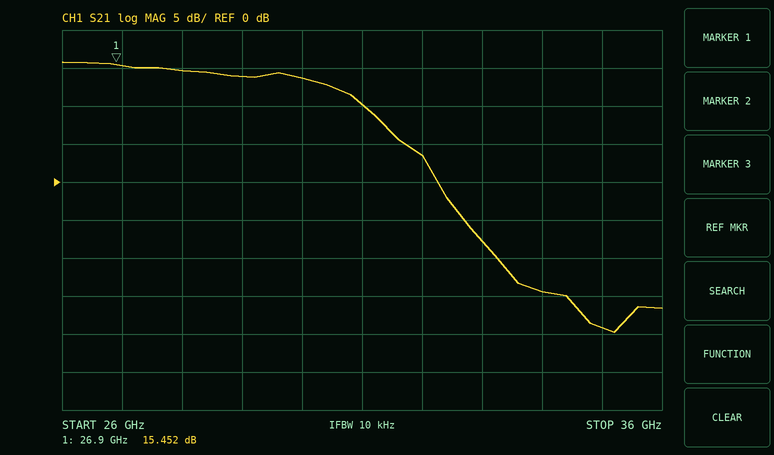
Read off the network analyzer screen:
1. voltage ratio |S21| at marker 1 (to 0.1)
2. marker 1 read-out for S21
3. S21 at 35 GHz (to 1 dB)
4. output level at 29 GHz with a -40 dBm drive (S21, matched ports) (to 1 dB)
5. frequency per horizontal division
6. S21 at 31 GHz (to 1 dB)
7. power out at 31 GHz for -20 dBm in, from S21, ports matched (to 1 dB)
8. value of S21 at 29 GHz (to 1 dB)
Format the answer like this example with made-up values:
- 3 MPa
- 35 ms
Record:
- 5.9
- 15.452 dB
- -19 dB
- -26 dBm
- 1 GHz
- 10 dB
- -10 dBm
- 14 dB
